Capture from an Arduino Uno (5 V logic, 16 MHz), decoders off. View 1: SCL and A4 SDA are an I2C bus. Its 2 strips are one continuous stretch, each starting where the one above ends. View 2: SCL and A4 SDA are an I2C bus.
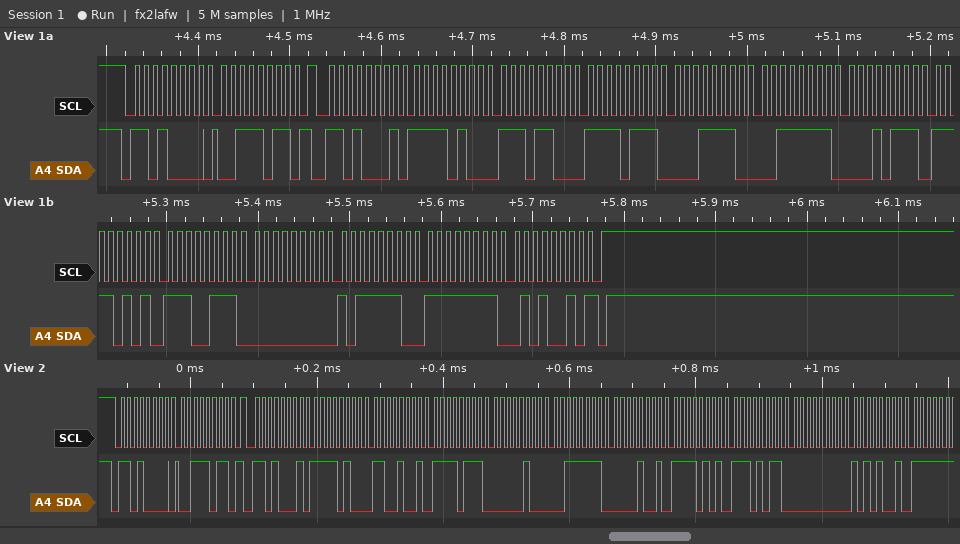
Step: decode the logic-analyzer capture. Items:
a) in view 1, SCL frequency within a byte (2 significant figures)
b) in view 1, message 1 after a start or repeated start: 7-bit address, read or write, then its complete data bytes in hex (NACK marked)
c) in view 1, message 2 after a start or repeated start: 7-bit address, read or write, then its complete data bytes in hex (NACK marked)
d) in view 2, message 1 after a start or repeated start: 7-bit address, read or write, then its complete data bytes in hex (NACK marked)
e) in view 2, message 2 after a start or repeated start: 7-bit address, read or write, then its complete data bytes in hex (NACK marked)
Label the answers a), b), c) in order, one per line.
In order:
a) 100 kHz
b) 0x68 write: 3B
c) 0x68 read: F4 EC F7 1E 3F 17 F5 E7 00 BE FF 52 NACK
d) 0x68 write: 3B
e) 0x68 read: F4 C9 F7 04 3F 09 F5 EB 00 A9
